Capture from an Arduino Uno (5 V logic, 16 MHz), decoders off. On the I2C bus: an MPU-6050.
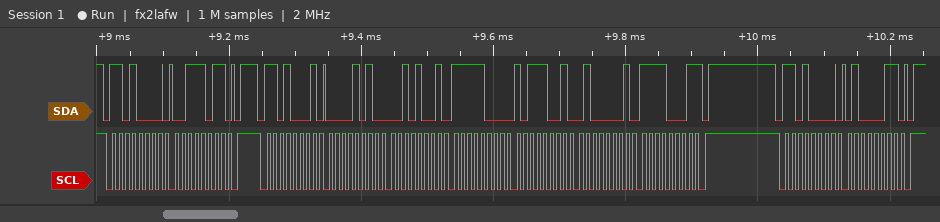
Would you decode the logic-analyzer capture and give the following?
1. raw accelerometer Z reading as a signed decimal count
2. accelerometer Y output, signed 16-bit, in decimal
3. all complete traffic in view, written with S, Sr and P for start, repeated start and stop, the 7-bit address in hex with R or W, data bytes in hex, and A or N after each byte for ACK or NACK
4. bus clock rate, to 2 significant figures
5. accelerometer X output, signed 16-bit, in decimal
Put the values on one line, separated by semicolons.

16881; -1863; S 68W A 3B A P S 68R A 0A A 29 A F8 A B9 A 41 A F1 N P S 68W A 43 A P; 100 kHz; 2601
